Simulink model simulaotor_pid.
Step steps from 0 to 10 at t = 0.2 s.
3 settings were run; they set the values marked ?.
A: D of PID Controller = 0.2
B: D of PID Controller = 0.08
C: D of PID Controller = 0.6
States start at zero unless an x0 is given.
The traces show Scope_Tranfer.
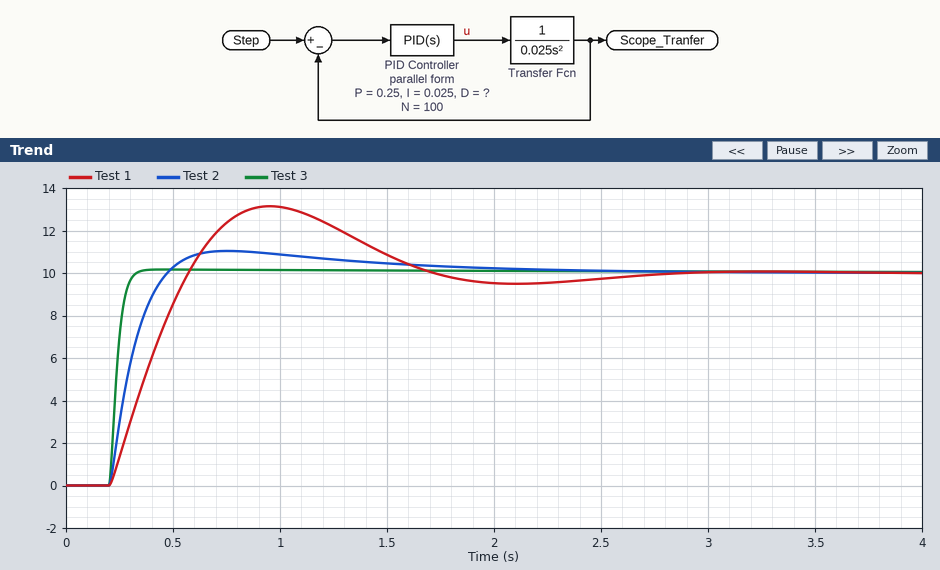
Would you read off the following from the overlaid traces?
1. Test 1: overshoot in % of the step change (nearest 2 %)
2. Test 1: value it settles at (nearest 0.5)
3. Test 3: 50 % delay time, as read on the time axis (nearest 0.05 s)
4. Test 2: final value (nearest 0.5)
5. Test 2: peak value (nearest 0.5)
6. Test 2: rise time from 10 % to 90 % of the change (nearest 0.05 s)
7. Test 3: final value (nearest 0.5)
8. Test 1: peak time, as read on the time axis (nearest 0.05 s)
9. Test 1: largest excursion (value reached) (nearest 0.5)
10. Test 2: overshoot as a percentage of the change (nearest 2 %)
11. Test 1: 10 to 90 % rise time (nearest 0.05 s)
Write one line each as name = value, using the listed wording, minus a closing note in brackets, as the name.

Test 1: overshoot in % of the step change = 32 %
Test 1: value it settles at = 10.0
Test 3: 50 % delay time, as read on the time axis = 0.25 s
Test 2: final value = 10.0
Test 2: peak value = 11.0
Test 2: rise time from 10 % to 90 % of the change = 0.20 s
Test 3: final value = 10.0
Test 1: peak time, as read on the time axis = 0.95 s
Test 1: largest excursion (value reached) = 13.0
Test 2: overshoot as a percentage of the change = 10 %
Test 1: 10 to 90 % rise time = 0.30 s
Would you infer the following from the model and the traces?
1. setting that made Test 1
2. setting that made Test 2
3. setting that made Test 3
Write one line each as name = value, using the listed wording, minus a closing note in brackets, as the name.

setting that made Test 1 = B
setting that made Test 2 = A
setting that made Test 3 = C
